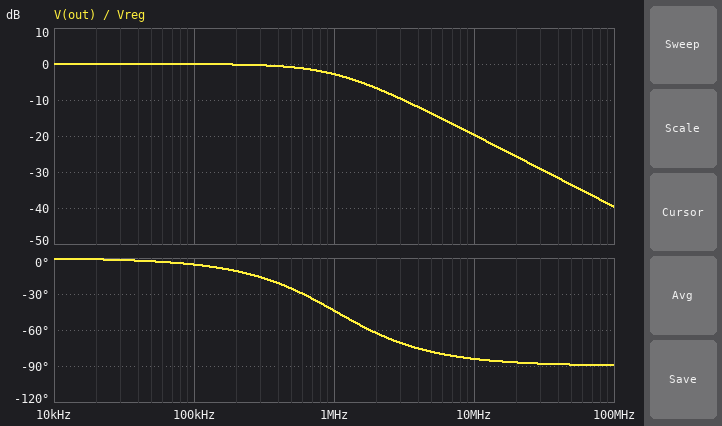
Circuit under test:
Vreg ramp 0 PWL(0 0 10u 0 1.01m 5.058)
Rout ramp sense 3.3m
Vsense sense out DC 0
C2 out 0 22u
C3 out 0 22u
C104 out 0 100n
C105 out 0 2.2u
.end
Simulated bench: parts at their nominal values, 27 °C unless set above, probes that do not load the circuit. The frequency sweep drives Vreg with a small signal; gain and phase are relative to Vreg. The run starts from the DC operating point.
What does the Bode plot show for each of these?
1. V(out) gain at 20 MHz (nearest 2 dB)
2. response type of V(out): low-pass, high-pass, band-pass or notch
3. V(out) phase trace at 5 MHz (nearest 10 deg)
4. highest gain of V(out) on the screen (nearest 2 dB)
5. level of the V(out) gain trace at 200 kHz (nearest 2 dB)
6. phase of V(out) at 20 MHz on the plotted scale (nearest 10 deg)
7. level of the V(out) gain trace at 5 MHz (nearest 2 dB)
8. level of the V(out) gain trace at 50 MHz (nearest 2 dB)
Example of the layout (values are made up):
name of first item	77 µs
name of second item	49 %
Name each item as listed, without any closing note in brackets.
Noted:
V(out) gain at 20 MHz	-26 dB
response type of V(out): low-pass, high-pass, band-pass or notch	low-pass
V(out) phase trace at 5 MHz	-80 deg
highest gain of V(out) on the screen	0 dB
level of the V(out) gain trace at 200 kHz	0 dB
phase of V(out) at 20 MHz on the plotted scale	-90 deg
level of the V(out) gain trace at 5 MHz	-14 dB
level of the V(out) gain trace at 50 MHz	-34 dB
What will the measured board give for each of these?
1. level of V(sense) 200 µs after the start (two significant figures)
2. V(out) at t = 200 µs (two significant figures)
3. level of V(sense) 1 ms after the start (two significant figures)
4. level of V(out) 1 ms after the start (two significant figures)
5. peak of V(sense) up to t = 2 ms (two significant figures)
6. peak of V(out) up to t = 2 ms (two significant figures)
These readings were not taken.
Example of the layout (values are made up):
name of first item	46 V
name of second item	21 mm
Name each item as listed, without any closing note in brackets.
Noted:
level of V(sense) 200 µs after the start	960 mV
V(out) at t = 200 µs	960 mV
level of V(sense) 1 ms after the start	5.0 V
level of V(out) 1 ms after the start	5.0 V
peak of V(sense) up to t = 2 ms	5.1 V
peak of V(out) up to t = 2 ms	5.1 V
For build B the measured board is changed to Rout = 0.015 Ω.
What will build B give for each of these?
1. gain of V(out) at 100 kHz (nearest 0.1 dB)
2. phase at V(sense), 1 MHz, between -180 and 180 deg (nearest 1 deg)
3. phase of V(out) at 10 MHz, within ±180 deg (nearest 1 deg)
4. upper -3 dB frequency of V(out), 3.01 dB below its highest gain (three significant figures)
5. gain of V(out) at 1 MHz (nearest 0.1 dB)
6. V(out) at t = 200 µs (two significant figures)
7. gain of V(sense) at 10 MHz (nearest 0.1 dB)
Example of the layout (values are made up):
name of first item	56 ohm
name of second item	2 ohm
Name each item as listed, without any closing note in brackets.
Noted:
gain of V(out) at 100 kHz	-0.8 dB
phase at V(sense), 1 MHz, between -180 and 180 deg	-77 deg
phase of V(out) at 10 MHz, within ±180 deg	-89 deg
upper -3 dB frequency of V(out), 3.01 dB below its highest gain	229 kHz
gain of V(out) at 1 MHz	-13.0 dB
V(out) at t = 200 µs	960 mV
gain of V(sense) at 10 MHz	-32.8 dB
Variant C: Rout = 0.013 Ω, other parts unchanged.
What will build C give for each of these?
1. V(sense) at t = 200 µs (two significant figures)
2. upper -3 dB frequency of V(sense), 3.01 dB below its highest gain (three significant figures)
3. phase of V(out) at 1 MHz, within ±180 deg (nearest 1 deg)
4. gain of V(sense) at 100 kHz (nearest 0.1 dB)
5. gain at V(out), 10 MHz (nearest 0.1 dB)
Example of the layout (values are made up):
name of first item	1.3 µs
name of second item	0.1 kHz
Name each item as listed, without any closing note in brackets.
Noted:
V(sense) at t = 200 µs	960 mV
upper -3 dB frequency of V(sense), 3.01 dB below its highest gain	264 kHz
phase of V(out) at 1 MHz, within ±180 deg	-75 deg
gain of V(sense) at 100 kHz	-0.6 dB
gain at V(out), 10 MHz	-31.6 dB
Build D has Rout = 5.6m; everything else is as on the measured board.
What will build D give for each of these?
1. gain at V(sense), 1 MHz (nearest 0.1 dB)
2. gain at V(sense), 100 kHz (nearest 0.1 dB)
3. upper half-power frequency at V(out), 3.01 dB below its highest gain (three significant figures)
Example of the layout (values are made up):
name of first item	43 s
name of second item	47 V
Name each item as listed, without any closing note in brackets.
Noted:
gain at V(sense), 1 MHz	-5.6 dB
gain at V(sense), 100 kHz	-0.1 dB
upper half-power frequency at V(out), 3.01 dB below its highest gain	614 kHz
